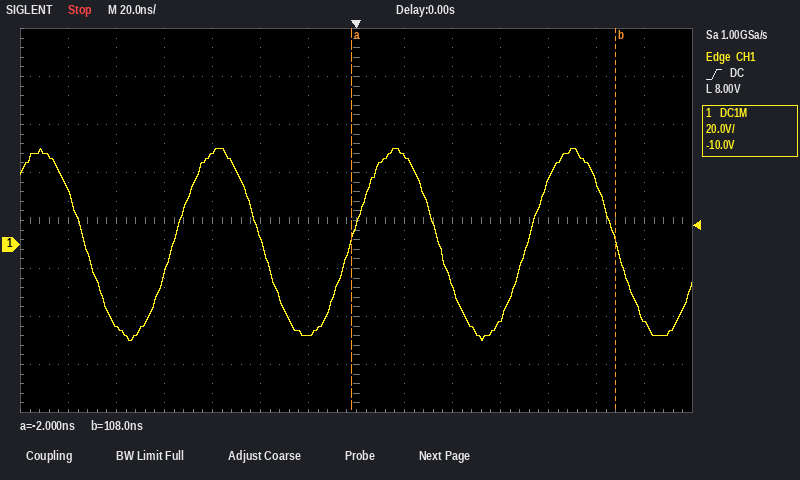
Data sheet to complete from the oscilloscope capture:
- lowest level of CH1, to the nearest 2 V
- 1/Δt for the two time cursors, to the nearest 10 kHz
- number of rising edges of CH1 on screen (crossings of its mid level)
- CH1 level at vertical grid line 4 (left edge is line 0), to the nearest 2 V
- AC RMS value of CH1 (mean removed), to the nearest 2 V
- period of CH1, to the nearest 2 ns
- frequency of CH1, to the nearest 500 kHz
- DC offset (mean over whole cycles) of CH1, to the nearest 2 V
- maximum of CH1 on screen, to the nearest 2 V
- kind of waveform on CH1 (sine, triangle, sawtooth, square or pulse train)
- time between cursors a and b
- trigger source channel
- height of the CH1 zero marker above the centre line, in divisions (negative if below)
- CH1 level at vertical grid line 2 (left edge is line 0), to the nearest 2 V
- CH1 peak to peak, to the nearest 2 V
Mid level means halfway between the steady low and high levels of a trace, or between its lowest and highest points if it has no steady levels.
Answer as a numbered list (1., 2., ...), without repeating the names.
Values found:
1. -40 V
2. 9.09 MHz
3. 3
4. 38 V
5. 28 V
6. 74 ns
7. 13.5 MHz
8. 0 V
9. 40 V
10. sine
11. 110 ns
12. CH1
13. -0.5 div
14. -34 V
15. 80 V
